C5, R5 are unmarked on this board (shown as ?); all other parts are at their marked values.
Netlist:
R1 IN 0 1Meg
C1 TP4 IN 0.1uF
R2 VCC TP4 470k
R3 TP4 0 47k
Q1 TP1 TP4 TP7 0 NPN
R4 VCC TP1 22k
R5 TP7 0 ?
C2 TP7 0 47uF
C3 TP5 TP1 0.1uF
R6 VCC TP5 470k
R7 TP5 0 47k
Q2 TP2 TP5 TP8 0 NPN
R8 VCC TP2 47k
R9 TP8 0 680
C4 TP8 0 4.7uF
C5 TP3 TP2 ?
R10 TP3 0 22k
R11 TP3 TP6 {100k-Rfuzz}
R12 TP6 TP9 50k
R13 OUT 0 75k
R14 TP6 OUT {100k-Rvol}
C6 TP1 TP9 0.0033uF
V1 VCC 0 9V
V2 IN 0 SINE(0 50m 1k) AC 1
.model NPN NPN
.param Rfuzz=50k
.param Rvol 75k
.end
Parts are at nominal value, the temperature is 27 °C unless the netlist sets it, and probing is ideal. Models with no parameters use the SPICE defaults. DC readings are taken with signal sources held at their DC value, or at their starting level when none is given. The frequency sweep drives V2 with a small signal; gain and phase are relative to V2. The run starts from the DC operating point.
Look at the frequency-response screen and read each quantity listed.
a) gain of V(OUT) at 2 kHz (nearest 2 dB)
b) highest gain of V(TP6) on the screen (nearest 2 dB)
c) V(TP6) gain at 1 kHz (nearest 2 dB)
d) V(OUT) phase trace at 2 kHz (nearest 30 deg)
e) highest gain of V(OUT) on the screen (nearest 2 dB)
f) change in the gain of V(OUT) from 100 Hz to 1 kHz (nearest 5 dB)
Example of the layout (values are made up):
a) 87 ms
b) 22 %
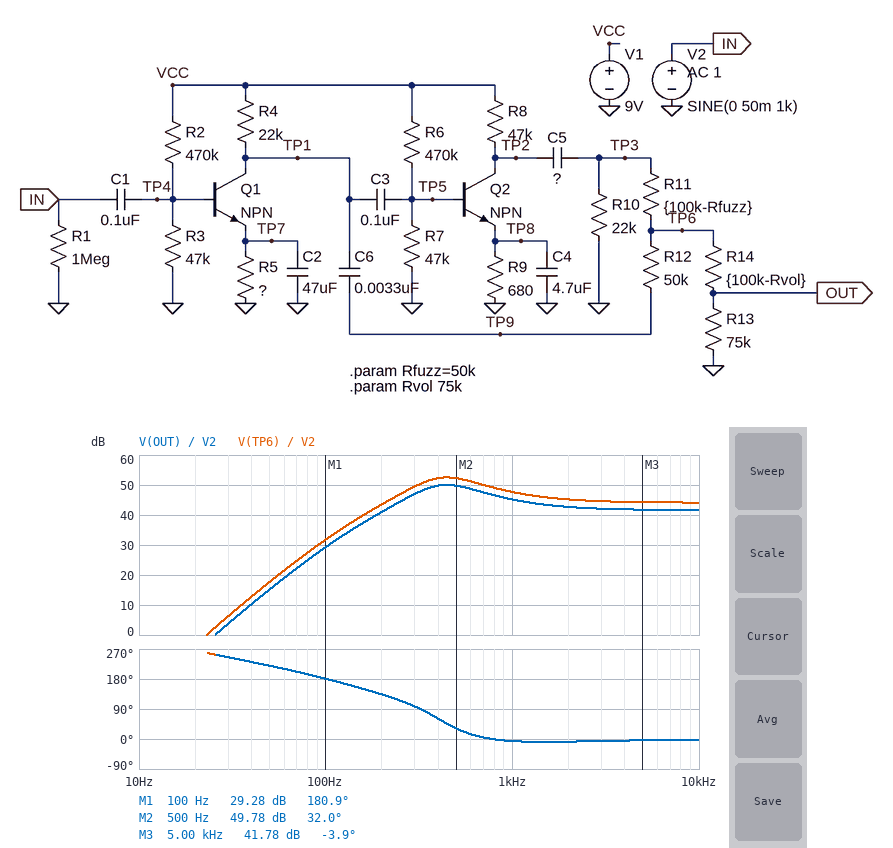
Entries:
a) 42 dB
b) 52 dB
c) 48 dB
d) 0 deg
e) 50 dB
f) 15 dB
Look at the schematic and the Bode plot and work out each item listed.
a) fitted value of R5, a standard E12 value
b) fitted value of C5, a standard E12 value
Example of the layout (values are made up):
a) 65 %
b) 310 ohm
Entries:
a) 470 Ω
b) 1.8 nF
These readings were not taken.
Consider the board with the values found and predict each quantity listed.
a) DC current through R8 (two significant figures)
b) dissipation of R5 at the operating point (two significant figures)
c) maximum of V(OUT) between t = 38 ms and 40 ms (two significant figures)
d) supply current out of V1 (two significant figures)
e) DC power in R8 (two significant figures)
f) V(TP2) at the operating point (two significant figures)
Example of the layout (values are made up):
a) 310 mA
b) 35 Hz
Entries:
a) 94 µA
b) 6.0 µW
c) 710 mV
d) 240 µA
e) 420 µW
f) 4.6 V
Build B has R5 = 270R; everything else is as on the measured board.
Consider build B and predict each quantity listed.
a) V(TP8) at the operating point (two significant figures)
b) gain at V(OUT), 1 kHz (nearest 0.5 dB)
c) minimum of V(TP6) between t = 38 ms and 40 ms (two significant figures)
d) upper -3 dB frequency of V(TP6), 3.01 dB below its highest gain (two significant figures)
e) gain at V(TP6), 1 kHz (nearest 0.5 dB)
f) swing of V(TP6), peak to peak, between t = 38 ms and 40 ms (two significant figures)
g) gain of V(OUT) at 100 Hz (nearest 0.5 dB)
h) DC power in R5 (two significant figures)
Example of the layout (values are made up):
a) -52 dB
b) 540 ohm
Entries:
a) 65 mV
b) 47.0 dB
c) -1.3 V
d) 760 Hz
e) 49.5 dB
f) 2.3 V
g) 30.0 dB
h) 5.1 µW
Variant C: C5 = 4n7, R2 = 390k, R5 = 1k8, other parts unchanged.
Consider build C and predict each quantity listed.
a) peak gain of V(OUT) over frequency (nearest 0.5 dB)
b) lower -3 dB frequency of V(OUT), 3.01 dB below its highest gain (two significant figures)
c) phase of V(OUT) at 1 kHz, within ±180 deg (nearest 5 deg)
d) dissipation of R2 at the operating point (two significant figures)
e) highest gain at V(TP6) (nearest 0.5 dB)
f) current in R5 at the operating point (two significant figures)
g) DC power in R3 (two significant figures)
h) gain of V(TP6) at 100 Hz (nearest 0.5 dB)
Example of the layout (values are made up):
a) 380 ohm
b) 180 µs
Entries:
a) 55.5 dB
b) 210 Hz
c) -20 deg
d) 170 µW
e) 58.0 dB
f) 110 µA
g) 18 µW
h) 40.5 dB
